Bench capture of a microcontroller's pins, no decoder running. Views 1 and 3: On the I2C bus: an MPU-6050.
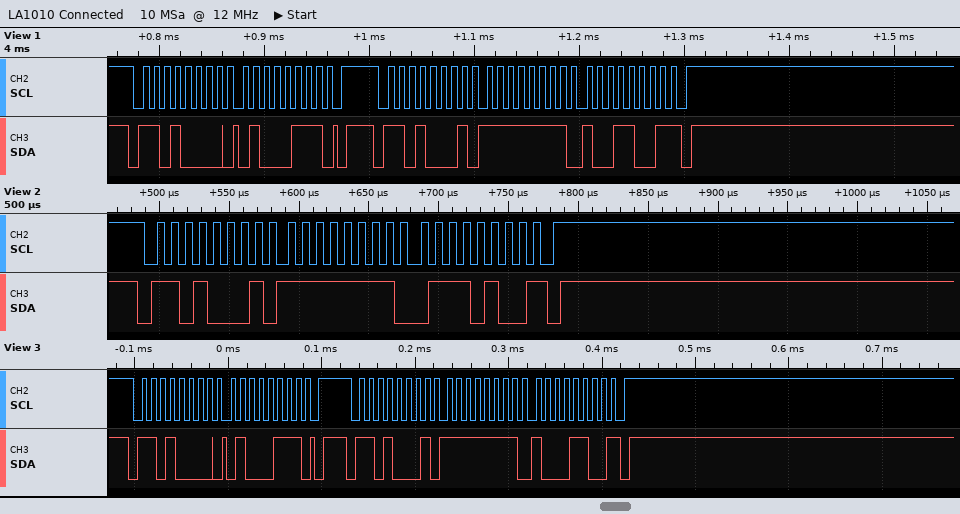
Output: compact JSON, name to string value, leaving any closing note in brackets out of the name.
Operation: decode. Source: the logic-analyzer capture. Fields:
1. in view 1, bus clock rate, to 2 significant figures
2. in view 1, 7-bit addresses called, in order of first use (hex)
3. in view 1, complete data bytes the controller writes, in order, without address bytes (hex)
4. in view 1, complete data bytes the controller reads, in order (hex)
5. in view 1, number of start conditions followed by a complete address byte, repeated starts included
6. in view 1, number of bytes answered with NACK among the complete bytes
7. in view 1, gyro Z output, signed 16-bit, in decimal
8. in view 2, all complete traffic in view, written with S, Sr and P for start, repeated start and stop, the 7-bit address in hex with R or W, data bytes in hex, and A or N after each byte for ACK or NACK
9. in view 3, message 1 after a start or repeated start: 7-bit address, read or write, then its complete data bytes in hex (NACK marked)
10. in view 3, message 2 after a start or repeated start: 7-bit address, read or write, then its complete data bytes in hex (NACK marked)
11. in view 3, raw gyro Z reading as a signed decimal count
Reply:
{"in view 1, bus clock rate, to 2 significant figures": "100 kHz", "in view 1, 7-bit addresses called, in order of first use": "0x68", "in view 1, complete data bytes the controller writes, in order, without address bytes": "47", "in view 1, complete data bytes the controller reads, in order": "FF 99", "in view 1, number of start conditions followed by a complete address byte, repeated starts included": "2", "in view 1, number of bytes answered with NACK among the complete bytes": "1", "in view 1, gyro Z output, signed 16-bit, in decimal": "-103", "in view 2, all complete traffic in view, written with S, Sr and P for start, repeated start and stop, the 7-bit address in hex with R or W, data bytes in hex, and A or N after each byte for ACK or NACK": "S 68R A FF A 74 N P", "in view 3, message 1 after a start or repeated start: 7-bit address, read or write, then its complete data bytes in hex": "0x68 write: 47", "in view 3, message 2 after a start or repeated start: 7-bit address, read or write, then its complete data bytes in hex": "0x68 read: FF 8C NACK", "in view 3, raw gyro Z reading as a signed decimal count": "-116"}
